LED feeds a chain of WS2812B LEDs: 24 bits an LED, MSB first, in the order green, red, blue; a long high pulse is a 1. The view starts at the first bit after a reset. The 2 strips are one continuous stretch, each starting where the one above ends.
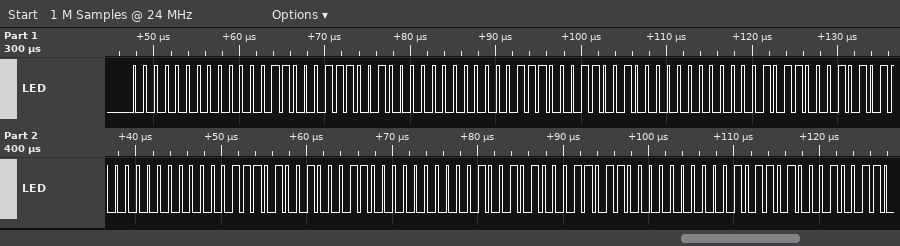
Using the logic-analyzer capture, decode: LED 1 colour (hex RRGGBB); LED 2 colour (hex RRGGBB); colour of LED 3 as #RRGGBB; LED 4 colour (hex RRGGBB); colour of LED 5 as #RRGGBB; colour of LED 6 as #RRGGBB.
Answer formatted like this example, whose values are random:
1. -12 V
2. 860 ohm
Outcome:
1. #060039
2. #0E0032
3. #16002A
4. #1D0023
5. #25001B
6. #2D0013
